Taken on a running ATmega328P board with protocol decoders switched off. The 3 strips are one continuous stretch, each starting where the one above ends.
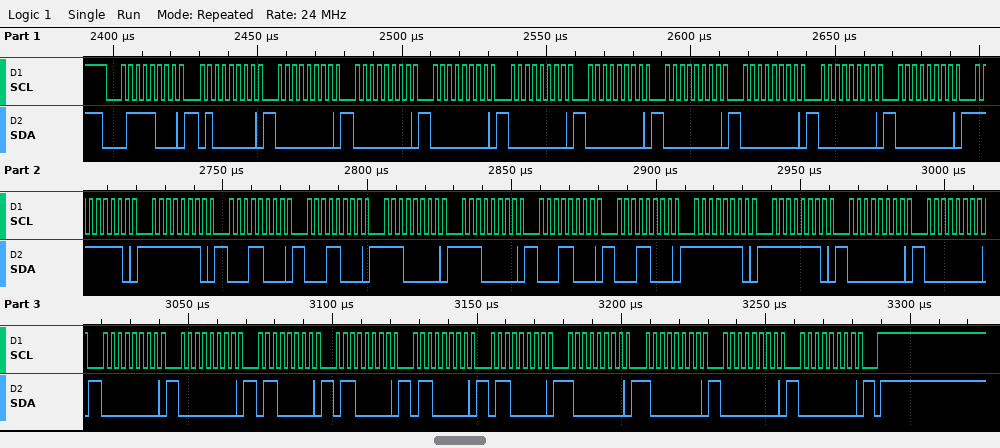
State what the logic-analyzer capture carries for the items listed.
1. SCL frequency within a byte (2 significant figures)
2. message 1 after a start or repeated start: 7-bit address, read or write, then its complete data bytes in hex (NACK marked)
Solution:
400 kHz
0x3C write: 40 00 00 00 00 00 00 00 00 00 FE FE 18 18 E0 E0 18 18 FE FE 00 00 00 00 60 60 60 60 80 80 00 00
